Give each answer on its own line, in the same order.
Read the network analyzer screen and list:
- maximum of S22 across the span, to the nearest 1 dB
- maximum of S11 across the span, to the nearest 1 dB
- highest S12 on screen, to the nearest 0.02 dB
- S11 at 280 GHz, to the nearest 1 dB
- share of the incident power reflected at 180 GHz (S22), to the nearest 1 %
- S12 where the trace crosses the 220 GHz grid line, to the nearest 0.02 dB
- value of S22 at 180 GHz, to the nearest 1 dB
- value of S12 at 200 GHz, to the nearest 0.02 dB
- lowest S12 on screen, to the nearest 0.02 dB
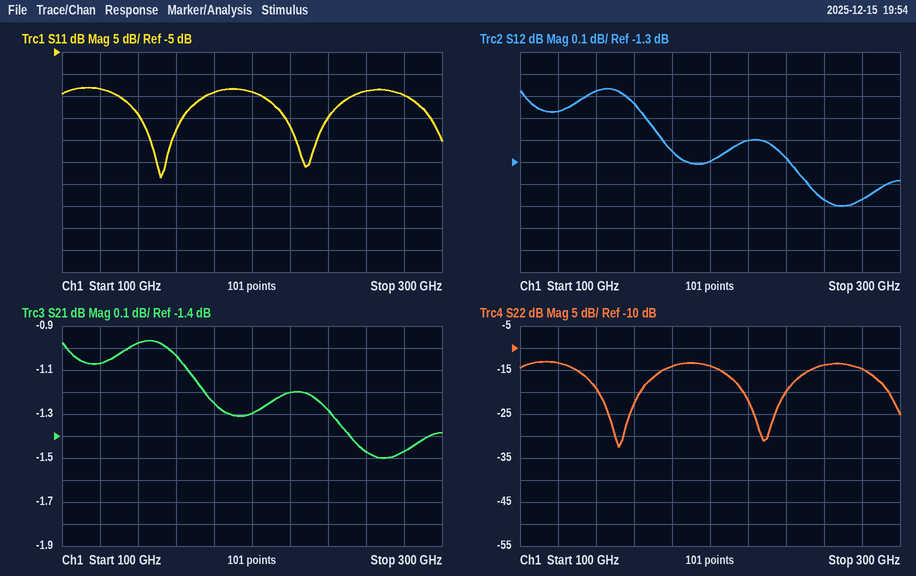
-13 dB
-13 dB
-0.96 dB
-15 dB
4 %
-1.20 dB
-14 dB
-1.30 dB
-1.50 dB
